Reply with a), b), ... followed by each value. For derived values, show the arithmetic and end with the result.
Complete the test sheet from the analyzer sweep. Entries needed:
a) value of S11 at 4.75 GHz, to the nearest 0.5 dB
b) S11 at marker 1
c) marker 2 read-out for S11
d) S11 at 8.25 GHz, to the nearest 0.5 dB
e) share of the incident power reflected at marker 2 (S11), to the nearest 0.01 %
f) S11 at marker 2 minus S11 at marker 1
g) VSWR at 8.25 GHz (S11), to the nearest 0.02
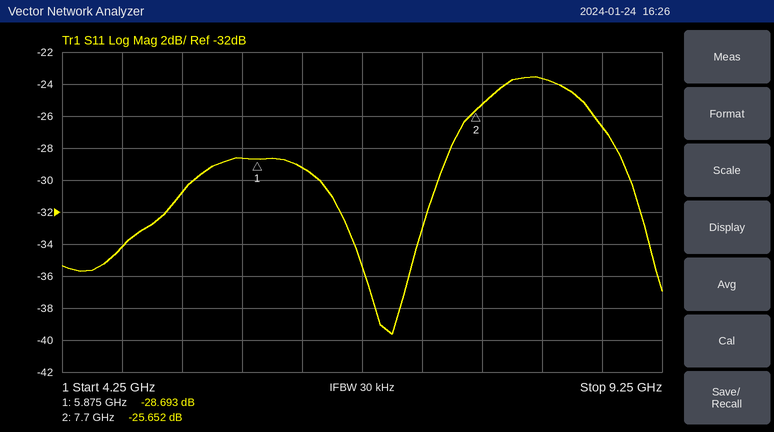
a) -34.0 dB
b) -28.693 dB
c) -25.652 dB
d) -23.5 dB
e) 10^(-25.652/10) ≈ 0.27 %
f) -25.652 − (-28.693) = 3.041 dB
g) |Γ| = 10^(-23.5/20) = 0.0668; VSWR = (1 + 0.0668)/(1 − 0.0668) ≈ 1.14
